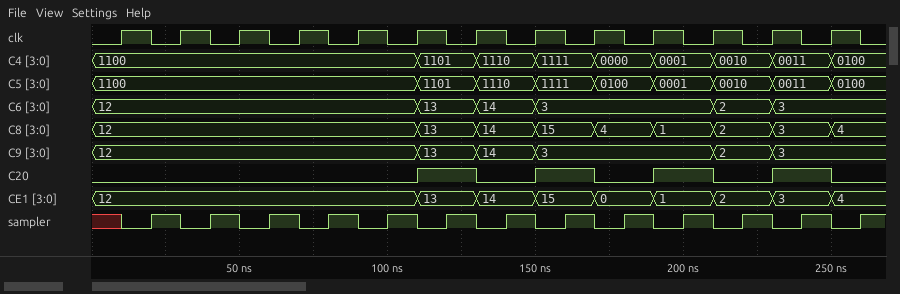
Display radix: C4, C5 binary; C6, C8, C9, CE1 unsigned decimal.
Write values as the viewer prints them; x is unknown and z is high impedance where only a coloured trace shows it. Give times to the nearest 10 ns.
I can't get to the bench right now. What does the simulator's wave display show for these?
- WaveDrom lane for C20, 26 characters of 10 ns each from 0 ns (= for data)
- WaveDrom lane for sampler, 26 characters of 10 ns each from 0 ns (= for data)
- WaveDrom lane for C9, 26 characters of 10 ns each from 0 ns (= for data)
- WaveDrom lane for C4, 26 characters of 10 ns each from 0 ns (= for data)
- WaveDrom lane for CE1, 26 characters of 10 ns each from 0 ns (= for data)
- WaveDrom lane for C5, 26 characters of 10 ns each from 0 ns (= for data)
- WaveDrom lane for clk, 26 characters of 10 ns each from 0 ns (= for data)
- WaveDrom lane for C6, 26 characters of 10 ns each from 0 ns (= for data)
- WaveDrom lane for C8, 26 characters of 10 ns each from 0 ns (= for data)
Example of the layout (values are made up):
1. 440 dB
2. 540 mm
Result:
1. {name: 'C20', wave: '0..........1.0.1.0.1.0.1.0'}
2. {name: 'sampler', wave: 'x0101010101010101010101010'}
3. {name: 'C9', wave: '=..........=.=.=.....=.=..', data: '12 13 14 3 2 3'}
4. {name: 'C4', wave: '=..........=.=.=.=.=.=.=.=', data: '1100 1101 1110 1111 0000 0001 0010 0011 0100'}
5. {name: 'CE1', wave: '=..........=.=.=.=.=.=.=.=', data: '12 13 14 15 0 1 2 3 4'}
6. {name: 'C5', wave: '=..........=.=.=.=.=.=.=.=', data: '1100 1101 1110 1111 0100 0001 0010 0011 0100'}
7. {name: 'clk', wave: '01010101010101010101010101'}
8. {name: 'C6', wave: '=..........=.=.=.....=.=..', data: '12 13 14 3 2 3'}
9. {name: 'C8', wave: '=..........=.=.=.=.=.=.=.=', data: '12 13 14 15 4 1 2 3 4'}
